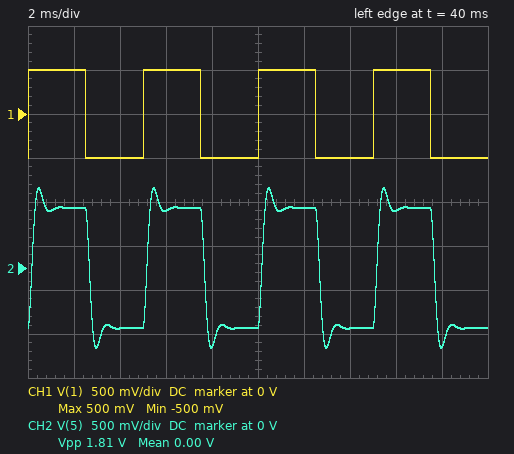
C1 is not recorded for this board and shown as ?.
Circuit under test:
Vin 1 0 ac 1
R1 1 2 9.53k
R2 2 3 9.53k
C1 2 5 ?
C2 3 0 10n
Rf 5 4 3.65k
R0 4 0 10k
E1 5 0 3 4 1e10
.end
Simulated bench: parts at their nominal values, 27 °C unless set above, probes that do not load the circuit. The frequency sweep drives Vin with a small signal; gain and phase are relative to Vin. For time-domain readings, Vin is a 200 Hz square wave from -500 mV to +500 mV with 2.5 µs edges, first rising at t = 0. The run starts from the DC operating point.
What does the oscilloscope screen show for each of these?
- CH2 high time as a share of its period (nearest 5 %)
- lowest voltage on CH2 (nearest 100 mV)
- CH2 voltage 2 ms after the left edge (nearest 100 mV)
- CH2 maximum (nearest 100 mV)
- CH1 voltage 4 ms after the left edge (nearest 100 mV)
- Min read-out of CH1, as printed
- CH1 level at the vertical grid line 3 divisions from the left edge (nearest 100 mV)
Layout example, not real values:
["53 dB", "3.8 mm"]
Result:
["50 %", "-900 mV", "700 mV", "900 mV", "-500 mV", "-500 mV", "500 mV"]
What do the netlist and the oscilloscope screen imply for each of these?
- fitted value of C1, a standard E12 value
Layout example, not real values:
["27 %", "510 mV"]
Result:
["18 nF"]
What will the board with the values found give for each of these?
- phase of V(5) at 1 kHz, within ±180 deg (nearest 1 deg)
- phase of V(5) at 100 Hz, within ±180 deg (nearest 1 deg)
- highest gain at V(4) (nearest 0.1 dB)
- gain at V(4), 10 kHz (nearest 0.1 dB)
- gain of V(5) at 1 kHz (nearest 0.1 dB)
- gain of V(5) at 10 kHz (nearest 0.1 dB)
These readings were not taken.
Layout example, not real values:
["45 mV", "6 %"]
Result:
["-66 deg", "-5 deg", "1.2 dB", "-36.1 dB", "3.8 dB", "-33.4 dB"]
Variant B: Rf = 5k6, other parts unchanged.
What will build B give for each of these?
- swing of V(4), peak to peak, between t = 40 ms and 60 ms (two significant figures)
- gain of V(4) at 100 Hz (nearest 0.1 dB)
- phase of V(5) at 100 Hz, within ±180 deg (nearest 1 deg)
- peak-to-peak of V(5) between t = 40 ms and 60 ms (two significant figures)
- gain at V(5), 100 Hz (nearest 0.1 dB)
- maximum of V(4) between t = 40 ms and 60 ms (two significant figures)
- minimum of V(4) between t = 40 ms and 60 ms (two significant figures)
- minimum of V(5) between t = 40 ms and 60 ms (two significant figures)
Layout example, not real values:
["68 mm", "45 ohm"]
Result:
["1.6 V", "0 dB", "-3 deg", "2.5 V", "3.9 dB", "790 mV", "-790 mV", "-1.2 V"]
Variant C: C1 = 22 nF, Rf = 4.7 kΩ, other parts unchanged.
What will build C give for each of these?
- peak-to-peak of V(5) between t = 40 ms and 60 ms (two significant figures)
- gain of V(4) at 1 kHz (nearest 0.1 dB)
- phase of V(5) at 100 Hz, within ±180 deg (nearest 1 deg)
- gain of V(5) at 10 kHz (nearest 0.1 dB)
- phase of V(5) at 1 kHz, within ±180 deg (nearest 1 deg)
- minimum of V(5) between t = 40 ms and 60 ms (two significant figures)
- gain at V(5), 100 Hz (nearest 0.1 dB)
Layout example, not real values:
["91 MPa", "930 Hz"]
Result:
["2.5 V", "4.2 dB", "-3 deg", "-34.5 dB", "-70 deg", "-1.2 V", "3.4 dB"]
